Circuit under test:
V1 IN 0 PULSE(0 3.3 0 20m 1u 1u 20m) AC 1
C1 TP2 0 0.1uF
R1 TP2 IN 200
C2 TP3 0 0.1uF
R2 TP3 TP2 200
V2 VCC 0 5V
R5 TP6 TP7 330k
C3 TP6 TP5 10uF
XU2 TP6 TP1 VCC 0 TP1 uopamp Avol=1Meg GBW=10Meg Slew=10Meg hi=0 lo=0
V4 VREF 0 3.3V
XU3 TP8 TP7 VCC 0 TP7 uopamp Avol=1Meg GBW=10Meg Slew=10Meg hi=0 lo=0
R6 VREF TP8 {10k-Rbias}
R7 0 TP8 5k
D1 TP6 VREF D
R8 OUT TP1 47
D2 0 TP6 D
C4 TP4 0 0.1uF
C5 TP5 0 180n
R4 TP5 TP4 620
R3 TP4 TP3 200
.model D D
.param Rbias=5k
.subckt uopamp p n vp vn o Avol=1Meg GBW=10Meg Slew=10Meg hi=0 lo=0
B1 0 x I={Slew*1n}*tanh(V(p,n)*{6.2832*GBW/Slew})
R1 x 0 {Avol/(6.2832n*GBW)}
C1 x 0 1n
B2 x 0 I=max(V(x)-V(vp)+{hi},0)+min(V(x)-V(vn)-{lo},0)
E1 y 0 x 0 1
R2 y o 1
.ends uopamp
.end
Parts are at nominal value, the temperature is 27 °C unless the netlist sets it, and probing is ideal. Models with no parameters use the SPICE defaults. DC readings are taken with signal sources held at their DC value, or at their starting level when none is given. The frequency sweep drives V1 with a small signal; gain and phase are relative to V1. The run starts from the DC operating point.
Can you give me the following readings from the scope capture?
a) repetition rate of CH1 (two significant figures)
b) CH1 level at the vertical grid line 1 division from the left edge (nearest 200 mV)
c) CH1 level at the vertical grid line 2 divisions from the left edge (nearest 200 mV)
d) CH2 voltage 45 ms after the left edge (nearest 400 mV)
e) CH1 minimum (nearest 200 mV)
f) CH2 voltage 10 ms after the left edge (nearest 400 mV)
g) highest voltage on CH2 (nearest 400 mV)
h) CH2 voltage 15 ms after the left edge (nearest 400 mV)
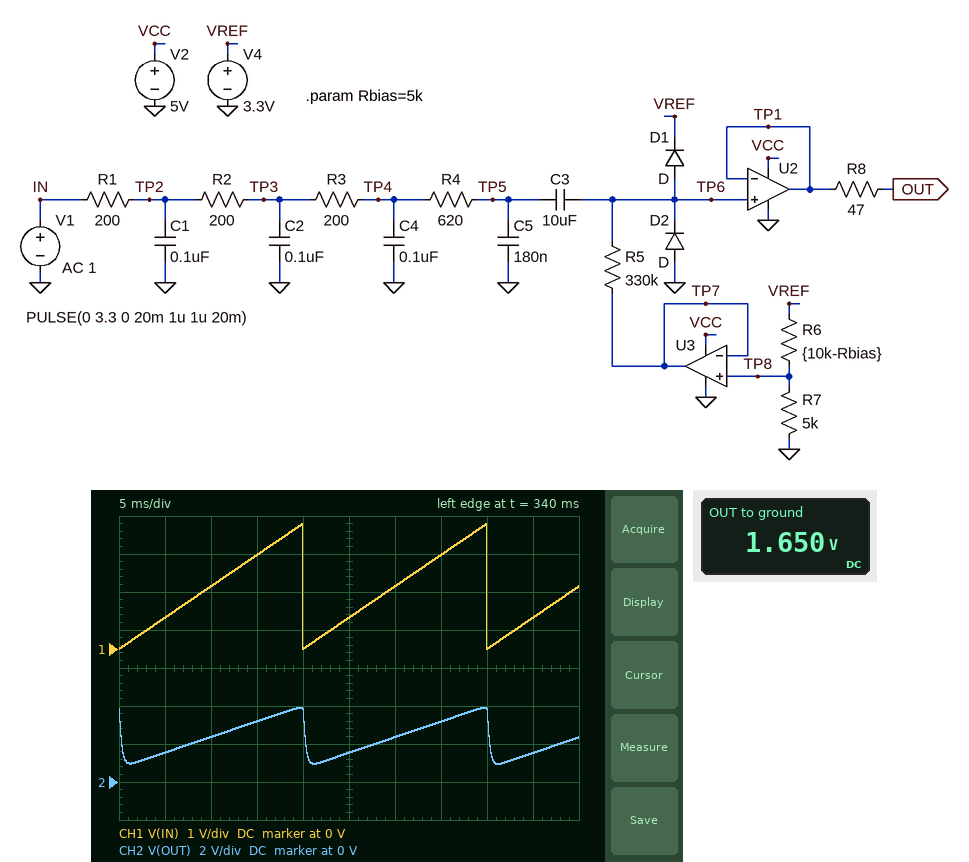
50 Hz
800 mV
1.6 V
1.6 V
0 V
2.4 V
4.0 V
3.2 V
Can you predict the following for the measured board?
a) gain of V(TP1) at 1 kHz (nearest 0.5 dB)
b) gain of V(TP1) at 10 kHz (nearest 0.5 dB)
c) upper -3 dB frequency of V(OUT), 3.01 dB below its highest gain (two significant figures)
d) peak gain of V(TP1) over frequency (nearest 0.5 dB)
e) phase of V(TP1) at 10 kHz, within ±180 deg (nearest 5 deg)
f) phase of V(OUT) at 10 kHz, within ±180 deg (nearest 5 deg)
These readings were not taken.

-6.5 dB
-37.0 dB
560 Hz
0 dB
145 deg
145 deg
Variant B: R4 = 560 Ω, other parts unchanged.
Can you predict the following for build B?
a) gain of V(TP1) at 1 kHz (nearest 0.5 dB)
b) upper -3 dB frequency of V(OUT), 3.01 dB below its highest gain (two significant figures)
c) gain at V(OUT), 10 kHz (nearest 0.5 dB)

-6.0 dB
580 Hz
-36.0 dB
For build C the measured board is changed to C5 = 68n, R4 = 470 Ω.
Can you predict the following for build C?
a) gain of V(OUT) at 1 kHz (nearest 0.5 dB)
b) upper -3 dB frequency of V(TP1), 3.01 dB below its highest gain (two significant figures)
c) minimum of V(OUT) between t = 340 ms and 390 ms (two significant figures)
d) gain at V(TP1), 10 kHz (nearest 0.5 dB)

-3.0 dB
1.0 kHz
850 mV
-27.5 dB
